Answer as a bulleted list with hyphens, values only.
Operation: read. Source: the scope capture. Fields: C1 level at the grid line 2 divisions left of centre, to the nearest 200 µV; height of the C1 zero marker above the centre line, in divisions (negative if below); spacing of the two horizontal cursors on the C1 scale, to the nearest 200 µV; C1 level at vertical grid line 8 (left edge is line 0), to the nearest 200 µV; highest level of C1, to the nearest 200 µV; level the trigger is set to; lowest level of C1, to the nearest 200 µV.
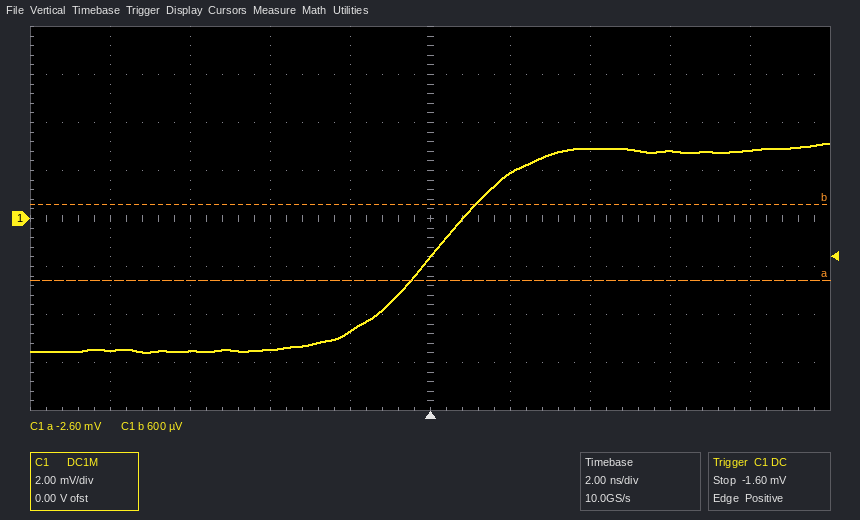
- -5.4 mV
- 0.0 div
- 3.2 mV
- 2.8 mV
- 3.2 mV
- -1.60 mV
- -5.6 mV
